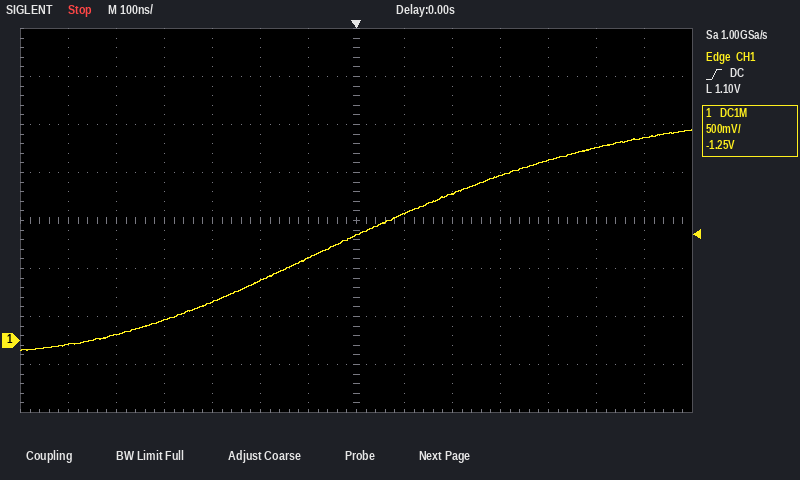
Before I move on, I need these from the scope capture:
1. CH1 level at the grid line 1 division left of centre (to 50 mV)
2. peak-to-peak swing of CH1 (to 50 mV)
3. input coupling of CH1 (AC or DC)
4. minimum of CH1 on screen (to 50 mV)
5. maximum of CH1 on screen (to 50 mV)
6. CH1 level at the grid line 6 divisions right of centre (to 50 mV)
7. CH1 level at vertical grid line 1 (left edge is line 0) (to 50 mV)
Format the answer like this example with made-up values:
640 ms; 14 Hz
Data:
850 mV; 2.30 V; DC; -100 mV; 2.20 V; 2.10 V; -50 mV
